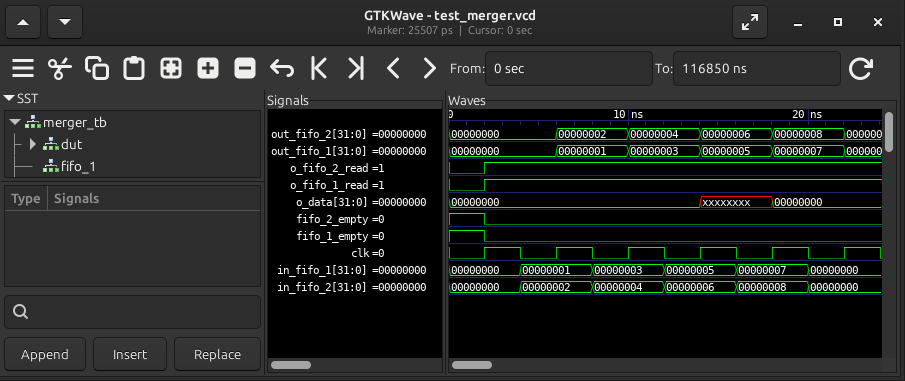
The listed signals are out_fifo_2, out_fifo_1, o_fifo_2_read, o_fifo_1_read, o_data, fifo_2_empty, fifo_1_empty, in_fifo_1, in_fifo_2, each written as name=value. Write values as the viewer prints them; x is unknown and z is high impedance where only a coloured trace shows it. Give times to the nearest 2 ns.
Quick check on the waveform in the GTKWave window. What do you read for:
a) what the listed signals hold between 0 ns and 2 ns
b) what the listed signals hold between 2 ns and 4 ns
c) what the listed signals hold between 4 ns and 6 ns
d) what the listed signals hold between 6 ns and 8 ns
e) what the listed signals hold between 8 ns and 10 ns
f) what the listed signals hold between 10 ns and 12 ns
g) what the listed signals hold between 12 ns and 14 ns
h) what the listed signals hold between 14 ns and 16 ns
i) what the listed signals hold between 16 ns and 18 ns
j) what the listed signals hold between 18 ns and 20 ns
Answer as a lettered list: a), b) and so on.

a) out_fifo_2=00000000, out_fifo_1=00000000, o_fifo_2_read=0, o_fifo_1_read=0, o_data=00000000, fifo_2_empty=1, fifo_1_empty=1, in_fifo_1=00000000, in_fifo_2=00000000
b) out_fifo_2=00000000, out_fifo_1=00000000, o_fifo_2_read=1, o_fifo_1_read=1, o_data=00000000, fifo_2_empty=0, fifo_1_empty=0, in_fifo_1=00000000, in_fifo_2=00000000
c) out_fifo_2=00000000, out_fifo_1=00000000, o_fifo_2_read=1, o_fifo_1_read=1, o_data=00000000, fifo_2_empty=0, fifo_1_empty=0, in_fifo_1=00000001, in_fifo_2=00000002
d) out_fifo_2=00000002, out_fifo_1=00000001, o_fifo_2_read=1, o_fifo_1_read=1, o_data=00000000, fifo_2_empty=0, fifo_1_empty=0, in_fifo_1=00000001, in_fifo_2=00000002
e) out_fifo_2=00000002, out_fifo_1=00000001, o_fifo_2_read=1, o_fifo_1_read=1, o_data=00000000, fifo_2_empty=0, fifo_1_empty=0, in_fifo_1=00000003, in_fifo_2=00000004
f) out_fifo_2=00000004, out_fifo_1=00000003, o_fifo_2_read=1, o_fifo_1_read=1, o_data=00000000, fifo_2_empty=0, fifo_1_empty=0, in_fifo_1=00000003, in_fifo_2=00000004
g) out_fifo_2=00000004, out_fifo_1=00000003, o_fifo_2_read=1, o_fifo_1_read=1, o_data=00000000, fifo_2_empty=0, fifo_1_empty=0, in_fifo_1=00000005, in_fifo_2=00000006
h) out_fifo_2=00000006, out_fifo_1=00000005, o_fifo_2_read=1, o_fifo_1_read=1, o_data=xxxxxxxx, fifo_2_empty=0, fifo_1_empty=0, in_fifo_1=00000005, in_fifo_2=00000006
i) out_fifo_2=00000006, out_fifo_1=00000005, o_fifo_2_read=1, o_fifo_1_read=1, o_data=xxxxxxxx, fifo_2_empty=0, fifo_1_empty=0, in_fifo_1=00000007, in_fifo_2=00000008
j) out_fifo_2=00000008, out_fifo_1=00000007, o_fifo_2_read=1, o_fifo_1_read=1, o_data=00000000, fifo_2_empty=0, fifo_1_empty=0, in_fifo_1=00000007, in_fifo_2=00000008
